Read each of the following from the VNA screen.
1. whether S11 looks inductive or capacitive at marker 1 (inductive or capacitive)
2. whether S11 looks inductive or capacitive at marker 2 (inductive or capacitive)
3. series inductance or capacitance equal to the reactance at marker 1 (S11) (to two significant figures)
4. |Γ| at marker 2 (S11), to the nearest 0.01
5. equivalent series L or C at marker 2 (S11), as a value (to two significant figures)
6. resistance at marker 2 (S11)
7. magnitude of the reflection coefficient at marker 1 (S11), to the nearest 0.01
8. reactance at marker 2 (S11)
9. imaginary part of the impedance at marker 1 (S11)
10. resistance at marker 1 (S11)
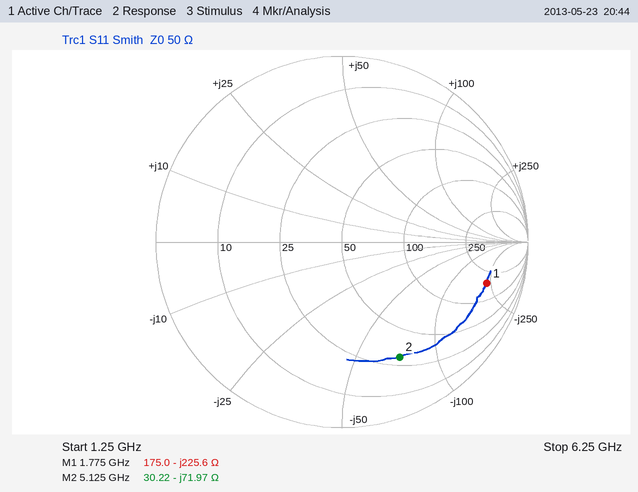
capacitive
capacitive
400 fF
0.69
430 fF
30.22 Ω
0.81
-71.97 Ω
-225.6 Ω
175.0 Ω
